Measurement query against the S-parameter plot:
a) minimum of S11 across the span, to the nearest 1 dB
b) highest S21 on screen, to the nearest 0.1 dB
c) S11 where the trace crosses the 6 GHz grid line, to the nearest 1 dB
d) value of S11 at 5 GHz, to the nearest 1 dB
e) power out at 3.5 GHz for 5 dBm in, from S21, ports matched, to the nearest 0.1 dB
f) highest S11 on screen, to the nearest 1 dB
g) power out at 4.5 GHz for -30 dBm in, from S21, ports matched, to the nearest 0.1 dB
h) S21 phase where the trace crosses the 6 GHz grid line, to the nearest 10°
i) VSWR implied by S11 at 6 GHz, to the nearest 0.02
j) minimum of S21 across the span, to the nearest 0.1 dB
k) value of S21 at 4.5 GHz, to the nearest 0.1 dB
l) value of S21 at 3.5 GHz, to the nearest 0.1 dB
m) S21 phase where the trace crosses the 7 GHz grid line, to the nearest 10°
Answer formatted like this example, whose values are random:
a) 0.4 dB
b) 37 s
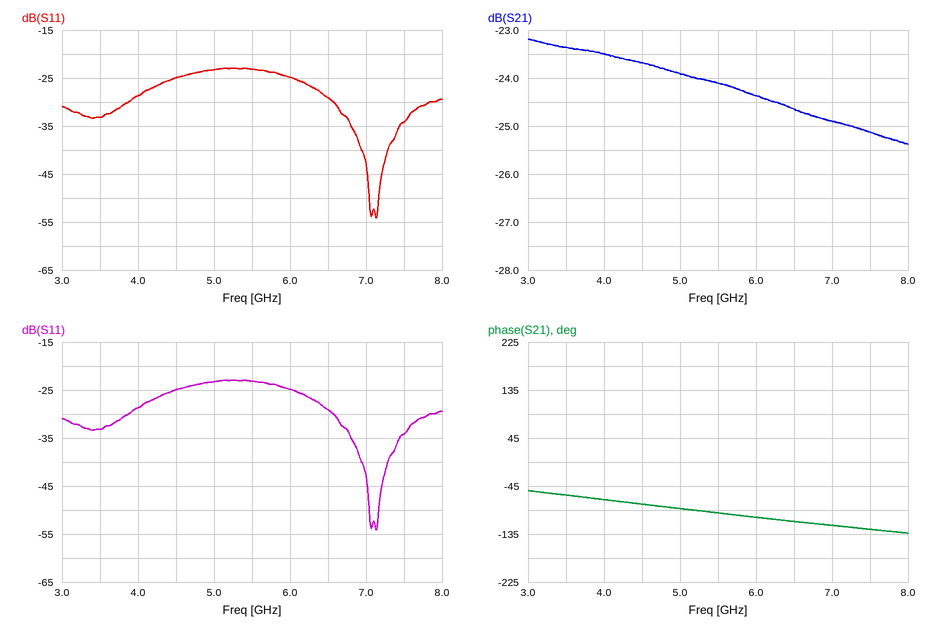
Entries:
a) -54 dB
b) -23.2 dB
c) -25 dB
d) -23 dB
e) -18.4 dBm
f) -23 dB
g) -53.7 dBm
h) -100°
i) 1.12
j) -25.4 dB
k) -23.7 dB
l) -23.4 dB
m) -120°
